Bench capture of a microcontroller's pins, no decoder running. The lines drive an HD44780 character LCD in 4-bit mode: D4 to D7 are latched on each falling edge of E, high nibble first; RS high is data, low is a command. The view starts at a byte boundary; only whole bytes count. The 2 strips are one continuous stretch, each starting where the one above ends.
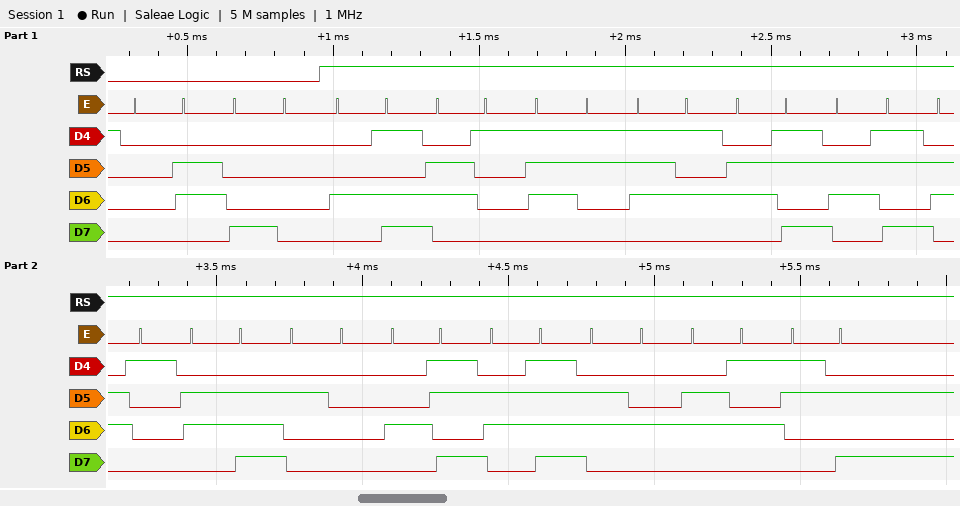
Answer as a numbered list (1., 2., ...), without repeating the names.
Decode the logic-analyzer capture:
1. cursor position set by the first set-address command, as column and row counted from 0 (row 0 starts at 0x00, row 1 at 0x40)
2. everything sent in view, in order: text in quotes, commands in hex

1. column 0, row 0
2. 0x06 0x80 "Masukkan Kode:"
